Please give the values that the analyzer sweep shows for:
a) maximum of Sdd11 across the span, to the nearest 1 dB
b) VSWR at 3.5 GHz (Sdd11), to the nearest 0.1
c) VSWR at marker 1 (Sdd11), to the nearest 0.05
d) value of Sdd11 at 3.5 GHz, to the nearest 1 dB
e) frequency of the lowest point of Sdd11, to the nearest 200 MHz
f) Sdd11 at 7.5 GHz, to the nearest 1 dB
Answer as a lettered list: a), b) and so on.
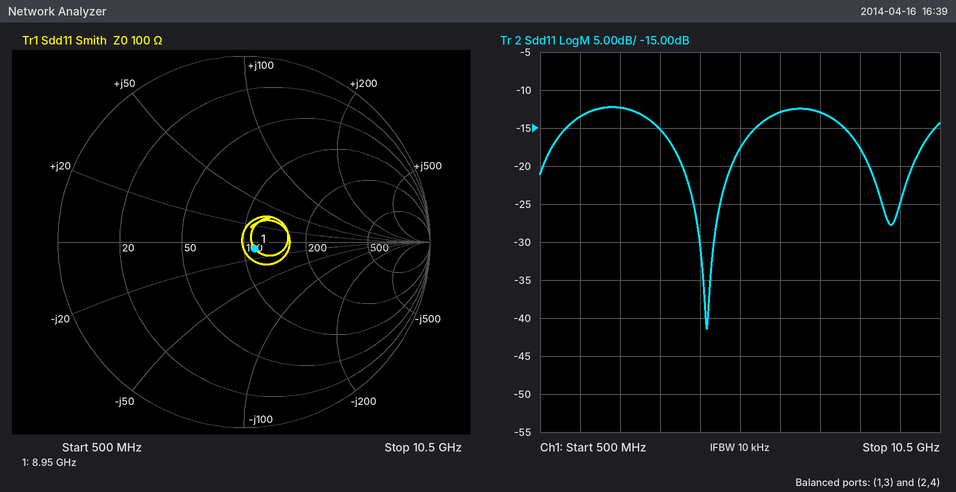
a) -12 dB
b) 1.4
c) 1.15
d) -15 dB
e) 4.6 GHz
f) -13 dB
